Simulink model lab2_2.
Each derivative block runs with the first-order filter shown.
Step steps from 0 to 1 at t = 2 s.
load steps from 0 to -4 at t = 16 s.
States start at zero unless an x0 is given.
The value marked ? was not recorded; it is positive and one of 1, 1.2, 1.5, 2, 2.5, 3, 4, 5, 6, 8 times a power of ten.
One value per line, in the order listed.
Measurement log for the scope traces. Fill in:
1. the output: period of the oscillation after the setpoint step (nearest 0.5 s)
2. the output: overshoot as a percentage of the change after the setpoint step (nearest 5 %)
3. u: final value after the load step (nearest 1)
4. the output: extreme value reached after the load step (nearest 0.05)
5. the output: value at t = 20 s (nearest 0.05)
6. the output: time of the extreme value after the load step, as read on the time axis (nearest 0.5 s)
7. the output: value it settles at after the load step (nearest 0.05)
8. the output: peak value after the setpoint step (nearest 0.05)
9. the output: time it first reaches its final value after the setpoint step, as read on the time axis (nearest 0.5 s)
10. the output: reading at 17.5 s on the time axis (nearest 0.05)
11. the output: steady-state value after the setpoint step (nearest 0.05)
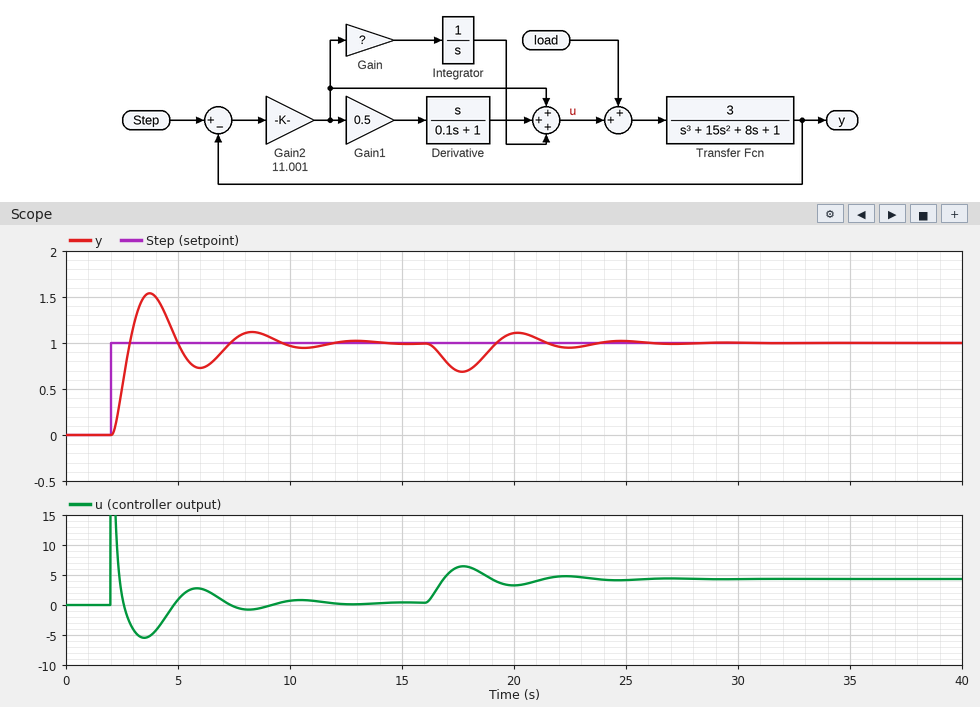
4.5 s
55 %
4
0.70
1.10
17.5 s
1.00
1.55
3.0 s
0.70
1.00
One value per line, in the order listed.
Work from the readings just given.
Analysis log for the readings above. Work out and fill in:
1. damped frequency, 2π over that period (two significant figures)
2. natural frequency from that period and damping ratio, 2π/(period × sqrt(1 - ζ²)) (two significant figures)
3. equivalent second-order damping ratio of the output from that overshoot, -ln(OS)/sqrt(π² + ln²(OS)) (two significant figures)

1.4 rad/s
1.4 rad/s
0.19
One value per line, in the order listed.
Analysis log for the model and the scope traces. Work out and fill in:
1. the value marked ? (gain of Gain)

0.8
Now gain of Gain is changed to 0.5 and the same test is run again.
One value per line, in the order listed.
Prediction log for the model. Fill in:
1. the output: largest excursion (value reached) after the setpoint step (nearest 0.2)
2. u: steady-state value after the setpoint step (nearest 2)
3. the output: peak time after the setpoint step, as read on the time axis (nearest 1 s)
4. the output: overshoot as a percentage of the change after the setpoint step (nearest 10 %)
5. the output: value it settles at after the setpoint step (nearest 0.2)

1.4
0
4 s
40 %
1.0
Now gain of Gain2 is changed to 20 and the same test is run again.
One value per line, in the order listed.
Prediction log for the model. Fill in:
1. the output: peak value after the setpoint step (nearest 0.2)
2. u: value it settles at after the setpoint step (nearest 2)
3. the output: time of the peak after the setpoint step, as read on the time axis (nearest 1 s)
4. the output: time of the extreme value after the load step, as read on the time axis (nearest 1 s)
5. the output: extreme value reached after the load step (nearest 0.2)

1.4
0
3 s
17 s
0.8
